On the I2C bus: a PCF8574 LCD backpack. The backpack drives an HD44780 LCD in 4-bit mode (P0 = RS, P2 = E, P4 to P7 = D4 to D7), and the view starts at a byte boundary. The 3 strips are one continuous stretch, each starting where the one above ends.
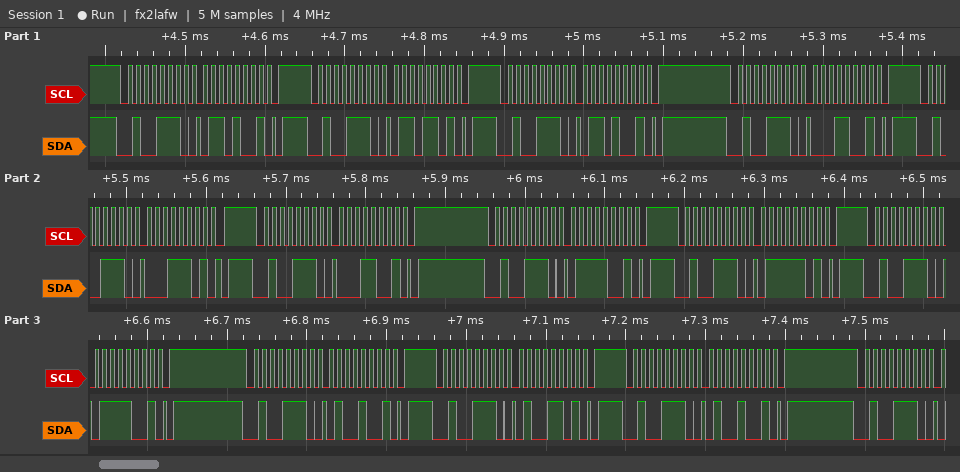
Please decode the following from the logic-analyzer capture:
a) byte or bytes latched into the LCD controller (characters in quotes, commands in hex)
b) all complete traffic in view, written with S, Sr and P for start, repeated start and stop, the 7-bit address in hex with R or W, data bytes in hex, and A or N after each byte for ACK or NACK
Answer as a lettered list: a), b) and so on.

a) 'a' 't'
b) S 27W A 69 A P S 27W A 6D A P S 27W A 69 A P S 27W A 19 A P S 27W A 1D A P S 27W A 19 A P S 27W A 79 A P S 27W A 7D A P S 27W A 79 A P S 27W A 49 A P S 27W A 4D A P S 27W A 49 A P S 27W A
